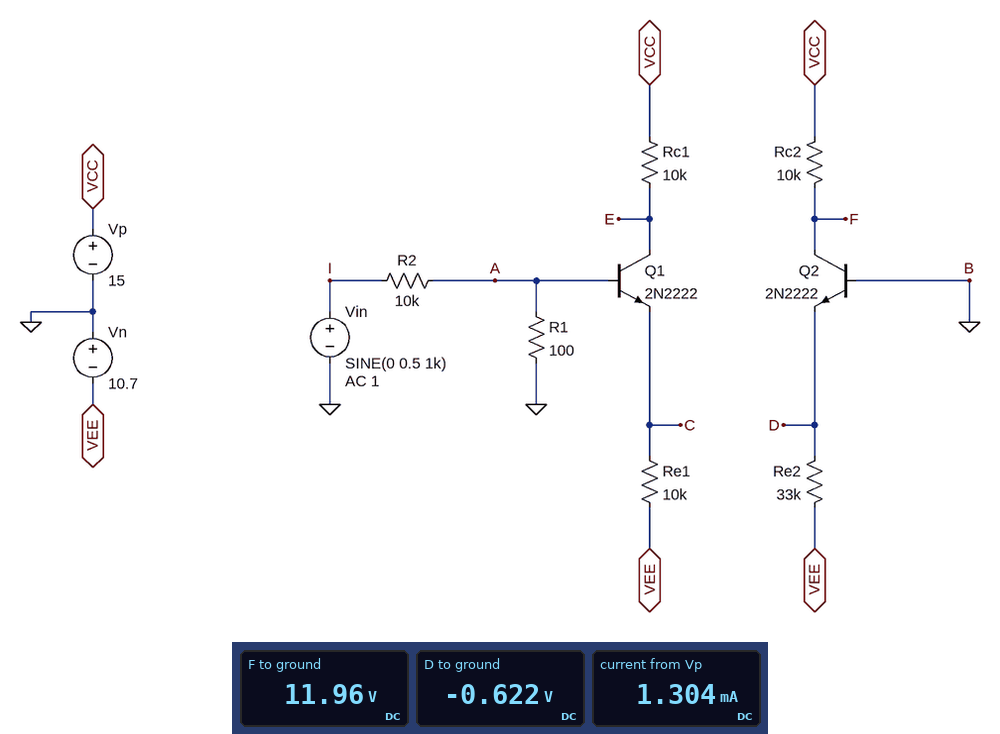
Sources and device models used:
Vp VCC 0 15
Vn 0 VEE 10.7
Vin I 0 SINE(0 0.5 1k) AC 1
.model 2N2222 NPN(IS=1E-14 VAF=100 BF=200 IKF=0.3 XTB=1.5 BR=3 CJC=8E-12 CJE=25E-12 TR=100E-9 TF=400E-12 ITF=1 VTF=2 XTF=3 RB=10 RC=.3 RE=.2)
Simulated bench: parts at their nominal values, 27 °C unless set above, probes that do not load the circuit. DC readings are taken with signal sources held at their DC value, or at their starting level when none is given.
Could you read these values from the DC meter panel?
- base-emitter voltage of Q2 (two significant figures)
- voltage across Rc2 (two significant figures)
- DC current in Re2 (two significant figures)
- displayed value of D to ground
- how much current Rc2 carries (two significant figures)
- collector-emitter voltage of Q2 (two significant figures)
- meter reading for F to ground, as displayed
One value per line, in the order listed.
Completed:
620 mV
3.0 V
310 µA
-0.622 V
300 µA
13 V
11.96 V
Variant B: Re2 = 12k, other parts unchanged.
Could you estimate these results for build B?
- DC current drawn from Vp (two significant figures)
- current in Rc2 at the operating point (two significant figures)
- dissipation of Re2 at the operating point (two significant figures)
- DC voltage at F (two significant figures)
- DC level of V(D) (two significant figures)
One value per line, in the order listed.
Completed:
1.8 mA
830 µA
8.4 mW
6.7 V
-650 mV
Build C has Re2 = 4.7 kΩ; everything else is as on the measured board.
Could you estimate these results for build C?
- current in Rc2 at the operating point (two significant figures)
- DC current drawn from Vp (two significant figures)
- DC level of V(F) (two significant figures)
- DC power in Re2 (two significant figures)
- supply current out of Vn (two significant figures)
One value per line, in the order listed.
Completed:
1.6 mA
2.6 mA
-670 mV
21 mW
3.1 mA
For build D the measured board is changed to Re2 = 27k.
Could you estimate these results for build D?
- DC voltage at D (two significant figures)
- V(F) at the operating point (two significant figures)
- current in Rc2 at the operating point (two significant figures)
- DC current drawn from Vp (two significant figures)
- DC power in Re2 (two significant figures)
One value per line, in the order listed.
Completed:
-630 mV
11 V
370 µA
1.4 mA
3.8 mW
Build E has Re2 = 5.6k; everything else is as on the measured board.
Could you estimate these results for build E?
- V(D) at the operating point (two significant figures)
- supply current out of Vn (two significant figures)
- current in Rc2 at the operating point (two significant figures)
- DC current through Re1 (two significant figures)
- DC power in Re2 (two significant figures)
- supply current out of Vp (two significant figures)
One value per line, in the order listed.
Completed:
-680 mV
2.8 mA
1.6 mA
1.0 mA
18 mW
2.6 mA
